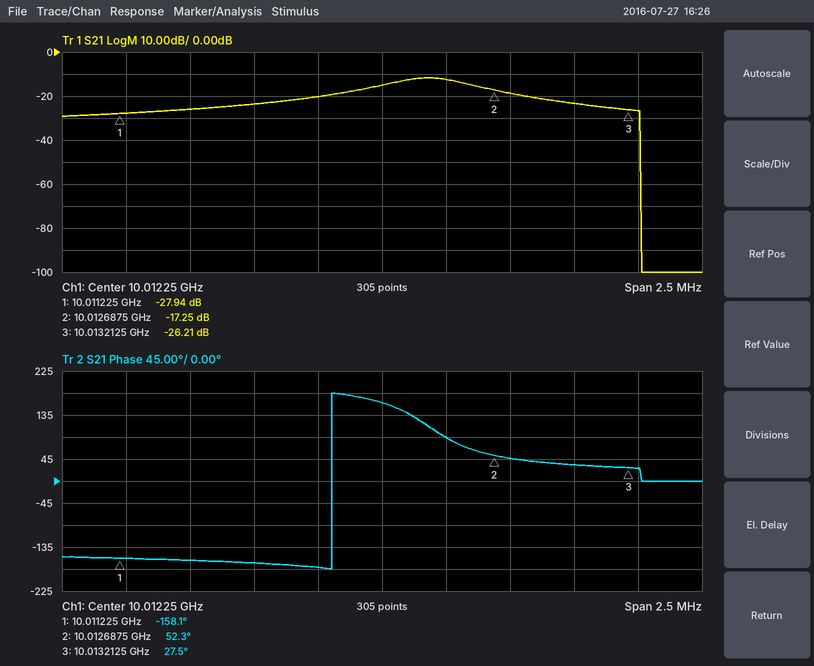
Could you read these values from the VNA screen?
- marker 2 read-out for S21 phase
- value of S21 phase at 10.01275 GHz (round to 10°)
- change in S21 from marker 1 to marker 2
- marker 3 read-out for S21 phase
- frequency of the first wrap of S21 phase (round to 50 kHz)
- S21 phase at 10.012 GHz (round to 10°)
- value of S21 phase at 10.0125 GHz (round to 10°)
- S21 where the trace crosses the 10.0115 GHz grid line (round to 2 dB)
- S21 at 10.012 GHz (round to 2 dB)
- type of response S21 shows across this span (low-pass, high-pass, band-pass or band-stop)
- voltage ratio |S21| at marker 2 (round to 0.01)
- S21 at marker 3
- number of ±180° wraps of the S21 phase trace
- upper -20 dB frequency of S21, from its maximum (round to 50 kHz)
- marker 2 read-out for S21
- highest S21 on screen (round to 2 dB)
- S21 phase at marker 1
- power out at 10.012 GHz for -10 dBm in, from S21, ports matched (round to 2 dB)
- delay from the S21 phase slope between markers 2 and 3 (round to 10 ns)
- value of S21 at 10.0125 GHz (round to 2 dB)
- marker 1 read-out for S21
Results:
52.3°
50°
10.69 dB
27.5°
10.01205 GHz
-180°
90°
-26 dB
-20 dB
band-pass
0.14
-26.21 dB
1
10.01325 GHz
-17.25 dB
-12 dB
-158.1°
-30 dBm
130 ns
-12 dB
-27.94 dB
